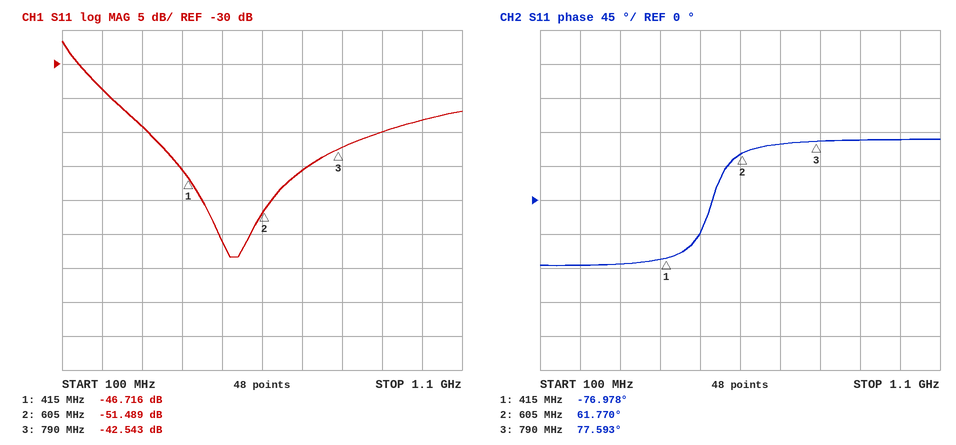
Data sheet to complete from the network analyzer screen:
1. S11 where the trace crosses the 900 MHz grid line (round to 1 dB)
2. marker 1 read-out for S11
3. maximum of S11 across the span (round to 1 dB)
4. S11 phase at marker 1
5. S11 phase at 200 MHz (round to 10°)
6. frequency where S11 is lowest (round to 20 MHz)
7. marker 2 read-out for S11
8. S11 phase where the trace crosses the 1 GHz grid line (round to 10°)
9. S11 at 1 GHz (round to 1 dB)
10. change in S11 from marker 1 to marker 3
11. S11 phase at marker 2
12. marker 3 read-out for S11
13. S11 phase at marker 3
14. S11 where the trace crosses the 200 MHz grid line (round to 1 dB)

-40 dB
-46.716 dB
-27 dB
-76.978°
-90°
520 MHz
-51.489 dB
80°
-38 dB
4.173 dB
61.770°
-42.543 dB
77.593°
-34 dB
